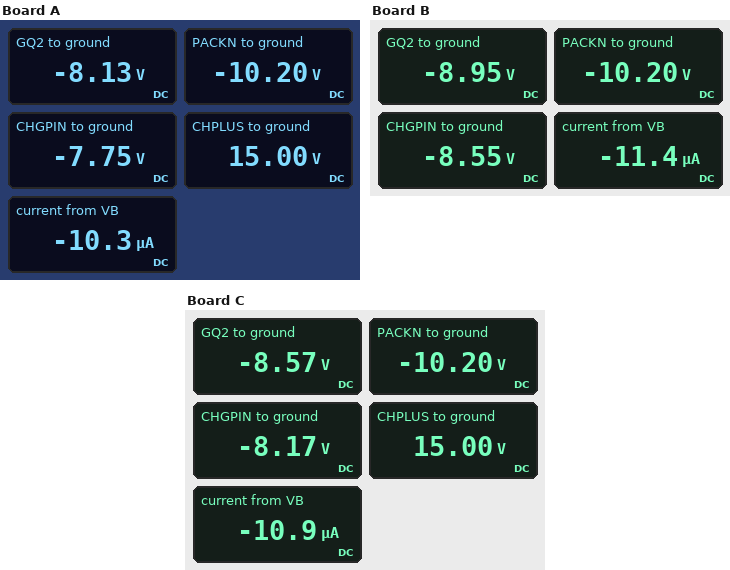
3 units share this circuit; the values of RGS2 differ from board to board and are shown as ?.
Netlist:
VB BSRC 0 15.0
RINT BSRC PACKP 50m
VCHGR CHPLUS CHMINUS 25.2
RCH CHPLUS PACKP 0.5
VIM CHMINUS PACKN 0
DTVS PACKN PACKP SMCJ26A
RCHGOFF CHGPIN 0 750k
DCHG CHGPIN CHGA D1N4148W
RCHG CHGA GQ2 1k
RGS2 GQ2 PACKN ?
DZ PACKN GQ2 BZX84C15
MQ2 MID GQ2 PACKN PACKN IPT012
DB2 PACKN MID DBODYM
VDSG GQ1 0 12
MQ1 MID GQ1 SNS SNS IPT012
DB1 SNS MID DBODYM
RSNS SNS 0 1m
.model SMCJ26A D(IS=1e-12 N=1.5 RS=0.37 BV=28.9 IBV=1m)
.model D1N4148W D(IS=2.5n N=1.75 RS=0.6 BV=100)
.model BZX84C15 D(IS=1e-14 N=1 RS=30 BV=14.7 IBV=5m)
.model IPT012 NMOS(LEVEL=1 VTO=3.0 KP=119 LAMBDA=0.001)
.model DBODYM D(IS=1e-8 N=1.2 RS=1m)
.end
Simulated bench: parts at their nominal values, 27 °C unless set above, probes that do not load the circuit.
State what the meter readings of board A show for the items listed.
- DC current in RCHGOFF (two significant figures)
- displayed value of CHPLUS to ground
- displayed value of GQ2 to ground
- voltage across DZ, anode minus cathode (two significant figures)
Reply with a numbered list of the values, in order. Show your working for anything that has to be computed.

1. (0 V - (-7.75 V)) / 750 kΩ = 10 µA
2. 15.00 V
3. -8.13 V
4. -10.2 V - (-8.13 V) = -2.1 V
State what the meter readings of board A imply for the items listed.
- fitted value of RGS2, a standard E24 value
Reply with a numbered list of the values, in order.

1. 200 kΩ
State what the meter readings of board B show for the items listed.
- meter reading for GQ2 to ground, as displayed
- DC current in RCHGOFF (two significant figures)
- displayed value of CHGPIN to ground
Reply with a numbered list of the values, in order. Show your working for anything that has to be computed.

1. -8.95 V
2. (0 V - (-8.55 V)) / 750 kΩ = 11 µA
3. -8.55 V
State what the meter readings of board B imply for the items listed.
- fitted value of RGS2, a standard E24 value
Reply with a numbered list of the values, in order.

1. 110 kΩ
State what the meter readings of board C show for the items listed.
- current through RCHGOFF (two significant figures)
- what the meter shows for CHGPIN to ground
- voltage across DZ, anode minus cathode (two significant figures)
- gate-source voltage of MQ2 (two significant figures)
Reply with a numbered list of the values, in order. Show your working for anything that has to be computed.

1. (0 V - (-8.17 V)) / 750 kΩ = 11 µA
2. -8.17 V
3. -10.2 V - (-8.57 V) = -1.6 V
4. -8.57 V - (-10.2 V) = 1.6 V
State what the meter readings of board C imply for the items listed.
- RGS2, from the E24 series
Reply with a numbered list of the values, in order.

1. 150 kΩ
